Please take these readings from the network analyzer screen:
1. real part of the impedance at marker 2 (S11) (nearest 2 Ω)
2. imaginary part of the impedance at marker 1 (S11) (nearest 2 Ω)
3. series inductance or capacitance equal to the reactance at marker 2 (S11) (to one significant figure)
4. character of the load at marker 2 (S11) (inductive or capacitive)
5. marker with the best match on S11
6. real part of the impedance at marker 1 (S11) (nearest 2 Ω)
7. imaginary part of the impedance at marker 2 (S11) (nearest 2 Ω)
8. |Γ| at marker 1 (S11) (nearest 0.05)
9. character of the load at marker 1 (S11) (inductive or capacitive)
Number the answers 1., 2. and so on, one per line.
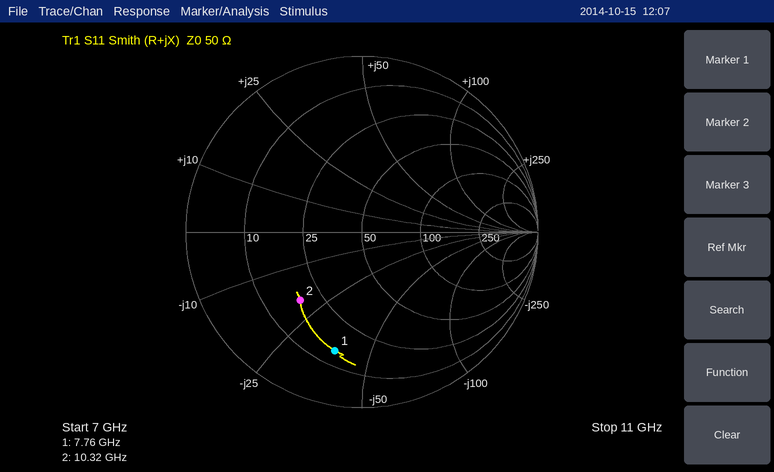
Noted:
1. 18 Ω
2. -38 Ω
3. 800 fF
4. capacitive
5. marker 2
6. 14 Ω
7. -20 Ω
8. 0.70
9. capacitive
